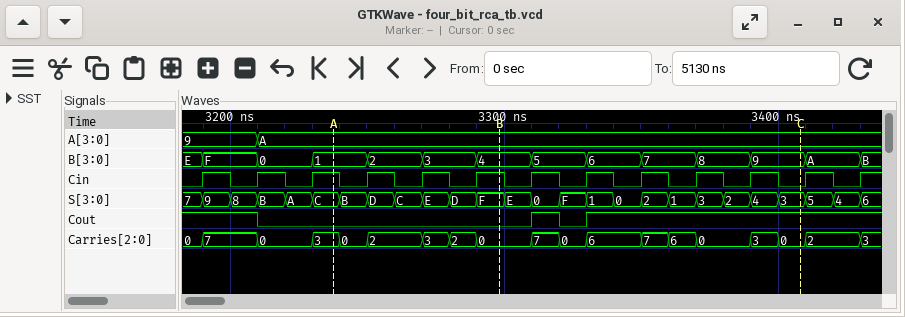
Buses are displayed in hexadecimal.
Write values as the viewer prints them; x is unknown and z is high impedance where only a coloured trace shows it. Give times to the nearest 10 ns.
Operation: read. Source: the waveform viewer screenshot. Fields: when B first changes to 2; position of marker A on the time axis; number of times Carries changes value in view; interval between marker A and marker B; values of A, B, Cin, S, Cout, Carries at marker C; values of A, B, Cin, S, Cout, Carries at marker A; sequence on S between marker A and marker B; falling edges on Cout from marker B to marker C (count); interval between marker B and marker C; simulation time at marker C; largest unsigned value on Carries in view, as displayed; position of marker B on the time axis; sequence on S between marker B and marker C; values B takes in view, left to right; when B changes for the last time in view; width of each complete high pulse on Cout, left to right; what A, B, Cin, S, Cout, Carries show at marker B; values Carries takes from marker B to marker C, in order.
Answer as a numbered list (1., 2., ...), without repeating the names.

1. 3250 ns
2. 3240 ns
3. 18
4. 60 ns
5. A=A, B=9, Cin=0, S=3, Cout=1, Carries=0
6. A=A, B=1, Cin=1, S=C, Cout=0, Carries=3
7. C, B, D, C, E, D, F
8. 1
9. 110 ns
10. 3410 ns
11. 7
12. 3300 ns
13. F, E, 0, F, 1, 0, 2, 1, 3, 2, 4, 3
14. E, F, 0, 1, 2, 3, 4, 5, 6, 7, 8, 9, A, B
15. 3430 ns
16. 10 ns
17. A=A, B=4, Cin=1, S=F, Cout=0, Carries=0
18. 0, 7, 0, 6, 7, 6, 0, 3, 0
